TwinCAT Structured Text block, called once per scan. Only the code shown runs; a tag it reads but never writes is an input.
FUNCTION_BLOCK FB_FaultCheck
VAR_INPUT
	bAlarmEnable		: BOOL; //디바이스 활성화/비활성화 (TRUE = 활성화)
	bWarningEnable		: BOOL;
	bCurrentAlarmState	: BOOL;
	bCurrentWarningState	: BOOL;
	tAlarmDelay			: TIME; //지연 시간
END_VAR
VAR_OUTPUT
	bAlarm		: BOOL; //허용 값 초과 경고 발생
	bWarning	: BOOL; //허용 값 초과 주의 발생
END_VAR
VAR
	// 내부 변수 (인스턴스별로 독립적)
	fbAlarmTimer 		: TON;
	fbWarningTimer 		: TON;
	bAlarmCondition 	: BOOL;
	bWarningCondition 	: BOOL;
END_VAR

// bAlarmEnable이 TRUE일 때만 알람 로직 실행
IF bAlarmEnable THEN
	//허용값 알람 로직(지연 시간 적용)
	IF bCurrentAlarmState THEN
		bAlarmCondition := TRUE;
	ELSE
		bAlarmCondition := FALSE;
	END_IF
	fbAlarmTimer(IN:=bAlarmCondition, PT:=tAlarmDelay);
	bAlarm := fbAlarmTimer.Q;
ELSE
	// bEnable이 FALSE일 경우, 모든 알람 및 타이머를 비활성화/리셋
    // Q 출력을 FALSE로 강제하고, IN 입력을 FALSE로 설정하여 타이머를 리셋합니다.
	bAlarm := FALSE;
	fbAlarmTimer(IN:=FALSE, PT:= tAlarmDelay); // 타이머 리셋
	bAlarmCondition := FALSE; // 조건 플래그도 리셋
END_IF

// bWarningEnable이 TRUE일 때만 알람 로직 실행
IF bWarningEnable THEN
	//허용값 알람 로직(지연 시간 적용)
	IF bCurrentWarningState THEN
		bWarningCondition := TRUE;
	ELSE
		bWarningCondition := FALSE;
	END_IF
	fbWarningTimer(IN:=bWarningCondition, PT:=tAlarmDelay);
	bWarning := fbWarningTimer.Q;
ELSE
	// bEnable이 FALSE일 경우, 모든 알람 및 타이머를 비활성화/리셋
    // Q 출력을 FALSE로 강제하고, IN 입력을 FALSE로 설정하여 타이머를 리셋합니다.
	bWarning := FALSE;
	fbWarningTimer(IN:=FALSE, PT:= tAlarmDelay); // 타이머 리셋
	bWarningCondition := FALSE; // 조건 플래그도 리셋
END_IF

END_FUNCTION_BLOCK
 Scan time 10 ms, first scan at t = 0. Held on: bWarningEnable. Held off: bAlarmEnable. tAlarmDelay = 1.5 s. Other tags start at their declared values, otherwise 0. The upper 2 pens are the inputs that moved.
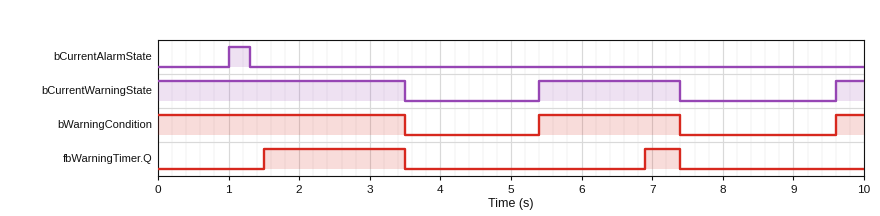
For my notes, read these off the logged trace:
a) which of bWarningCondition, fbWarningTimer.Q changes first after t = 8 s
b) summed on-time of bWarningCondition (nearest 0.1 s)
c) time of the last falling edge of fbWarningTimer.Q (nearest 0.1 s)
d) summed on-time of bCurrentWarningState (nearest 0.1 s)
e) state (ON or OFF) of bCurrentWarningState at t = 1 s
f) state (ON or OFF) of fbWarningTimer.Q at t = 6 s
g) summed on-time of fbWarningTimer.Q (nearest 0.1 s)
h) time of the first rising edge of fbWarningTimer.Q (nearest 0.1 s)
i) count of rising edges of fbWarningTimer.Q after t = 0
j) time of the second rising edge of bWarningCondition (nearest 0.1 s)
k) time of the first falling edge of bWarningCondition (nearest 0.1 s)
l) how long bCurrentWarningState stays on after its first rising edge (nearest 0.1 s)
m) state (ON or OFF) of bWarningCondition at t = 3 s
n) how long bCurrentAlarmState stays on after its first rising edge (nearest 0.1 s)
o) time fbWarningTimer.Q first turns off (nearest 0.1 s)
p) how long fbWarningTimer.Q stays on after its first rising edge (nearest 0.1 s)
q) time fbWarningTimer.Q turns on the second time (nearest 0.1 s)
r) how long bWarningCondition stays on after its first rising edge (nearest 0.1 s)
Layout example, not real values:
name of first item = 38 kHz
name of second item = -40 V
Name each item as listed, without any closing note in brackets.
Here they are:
which of bWarningCondition, fbWarningTimer.Q changes first after t = 8 s = bWarningCondition
summed on-time of bWarningCondition = 5.9 s
time of the last falling edge of fbWarningTimer.Q = 7.4 s
summed on-time of bCurrentWarningState = 5.9 s
state (ON or OFF) of bCurrentWarningState at t = 1 s = ON
state (ON or OFF) of fbWarningTimer.Q at t = 6 s = OFF
summed on-time of fbWarningTimer.Q = 2.5 s
time of the first rising edge of fbWarningTimer.Q = 1.5 s
count of rising edges of fbWarningTimer.Q after t = 0 = 2
time of the second rising edge of bWarningCondition = 9.6 s
time of the first falling edge of bWarningCondition = 3.5 s
how long bCurrentWarningState stays on after its first rising edge = 2.0 s
state (ON or OFF) of bWarningCondition at t = 3 s = ON
how long bCurrentAlarmState stays on after its first rising edge = 0.3 s
time fbWarningTimer.Q first turns off = 3.5 s
how long fbWarningTimer.Q stays on after its first rising edge = 2.0 s
time fbWarningTimer.Q turns on the second time = 6.9 s
how long bWarningCondition stays on after its first rising edge = 2.0 s
